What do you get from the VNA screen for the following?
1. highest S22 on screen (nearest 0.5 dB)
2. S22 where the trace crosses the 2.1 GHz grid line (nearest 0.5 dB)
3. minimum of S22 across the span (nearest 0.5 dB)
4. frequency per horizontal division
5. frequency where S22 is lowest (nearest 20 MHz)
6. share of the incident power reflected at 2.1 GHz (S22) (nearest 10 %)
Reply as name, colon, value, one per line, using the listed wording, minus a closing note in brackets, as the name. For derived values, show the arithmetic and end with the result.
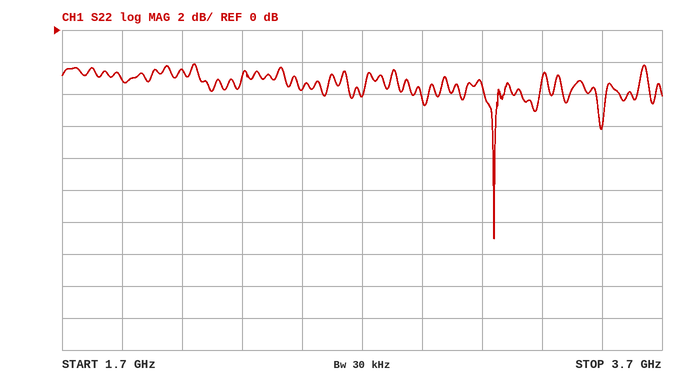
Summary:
highest S22 on screen: -2.0 dB
S22 where the trace crosses the 2.1 GHz grid line: -2.5 dB
minimum of S22 across the span: -13.0 dB
frequency per horizontal division: 200 MHz
frequency where S22 is lowest: 3.14 GHz
share of the incident power reflected at 2.1 GHz (S22): 10^(-2.5/10) ≈ 56.2 %, so 60 % to the nearest 10 %
